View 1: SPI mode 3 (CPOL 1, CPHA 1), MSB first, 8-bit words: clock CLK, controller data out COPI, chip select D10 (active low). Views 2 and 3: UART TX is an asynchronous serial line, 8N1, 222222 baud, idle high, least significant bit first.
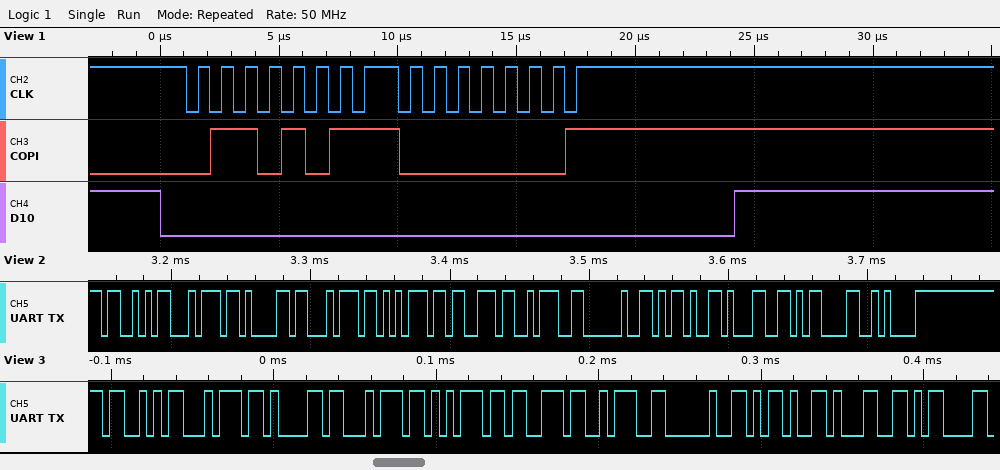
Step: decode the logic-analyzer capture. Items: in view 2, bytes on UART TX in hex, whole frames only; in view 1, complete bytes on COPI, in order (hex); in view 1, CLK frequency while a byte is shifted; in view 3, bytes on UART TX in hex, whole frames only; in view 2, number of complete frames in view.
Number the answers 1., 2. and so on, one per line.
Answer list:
1. 0x53 0x74 0x61 0x74 0x75 0x73 0x3A 0x20 0x2D 0x31 0x0D 0x0A
2. 6B 01
3. 1 MHz
4. 53 74 61 74 75 73 3A 20 2D 31 0D
5. 12
